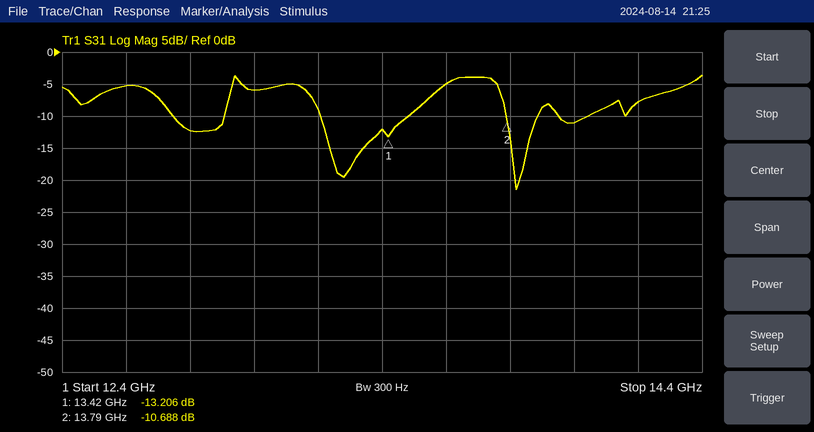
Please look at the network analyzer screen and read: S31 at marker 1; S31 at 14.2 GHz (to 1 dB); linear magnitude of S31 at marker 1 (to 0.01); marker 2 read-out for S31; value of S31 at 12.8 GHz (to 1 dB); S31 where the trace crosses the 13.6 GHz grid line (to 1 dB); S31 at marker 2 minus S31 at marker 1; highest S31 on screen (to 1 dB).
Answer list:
-13.206 dB
-8 dB
0.22
-10.688 dB
-12 dB
-5 dB
2.518 dB
-4 dB
